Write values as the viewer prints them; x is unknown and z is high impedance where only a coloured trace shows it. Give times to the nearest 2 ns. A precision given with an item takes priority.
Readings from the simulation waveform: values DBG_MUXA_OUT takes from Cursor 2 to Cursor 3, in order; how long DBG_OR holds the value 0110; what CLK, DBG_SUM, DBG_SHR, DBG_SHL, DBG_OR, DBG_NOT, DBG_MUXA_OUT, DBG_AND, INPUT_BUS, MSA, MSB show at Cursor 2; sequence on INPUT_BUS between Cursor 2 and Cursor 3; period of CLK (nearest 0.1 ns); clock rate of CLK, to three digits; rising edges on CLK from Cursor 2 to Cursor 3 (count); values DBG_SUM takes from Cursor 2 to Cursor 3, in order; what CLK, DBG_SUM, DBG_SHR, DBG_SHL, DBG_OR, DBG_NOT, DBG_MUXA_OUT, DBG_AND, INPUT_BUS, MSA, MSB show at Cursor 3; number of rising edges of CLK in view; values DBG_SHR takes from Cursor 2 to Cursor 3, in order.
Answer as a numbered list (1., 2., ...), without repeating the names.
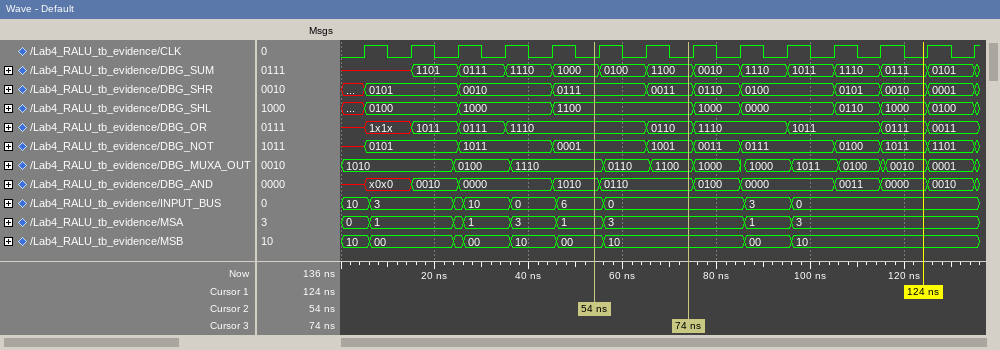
1. 1110, 0110, 1100
2. 10 ns
3. CLK=0, DBG_SUM=1000, DBG_SHR=0111, DBG_SHL=1100, DBG_OR=1110, DBG_NOT=0001, DBG_MUXA_OUT=1110, DBG_AND=1010, INPUT_BUS=6, MSA=1, MSB=00
4. 6, 0
5. 10 ns
6. 100 MHz
7. 2
8. 1000, 0100, 1100
9. CLK=0, DBG_SUM=1100, DBG_SHR=0011, DBG_SHL=1100, DBG_OR=0110, DBG_NOT=1001, DBG_MUXA_OUT=1100, DBG_AND=0110, INPUT_BUS=0, MSA=3, MSB=10
10. 14
11. 0111, 0011
